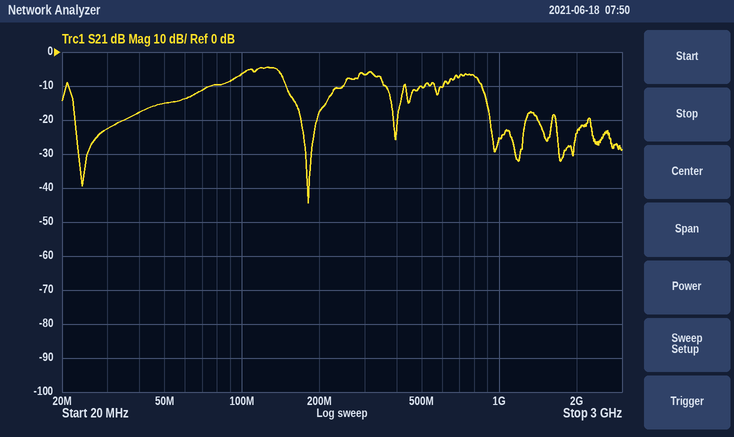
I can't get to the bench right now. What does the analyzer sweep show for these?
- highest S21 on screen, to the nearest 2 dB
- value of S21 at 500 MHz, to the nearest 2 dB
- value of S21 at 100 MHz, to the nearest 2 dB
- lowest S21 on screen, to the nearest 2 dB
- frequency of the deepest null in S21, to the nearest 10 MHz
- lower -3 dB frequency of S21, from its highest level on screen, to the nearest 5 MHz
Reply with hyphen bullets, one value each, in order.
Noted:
- -4 dB
- -10 dB
- -6 dB
- -44 dB
- 180 MHz
- 95 MHz
